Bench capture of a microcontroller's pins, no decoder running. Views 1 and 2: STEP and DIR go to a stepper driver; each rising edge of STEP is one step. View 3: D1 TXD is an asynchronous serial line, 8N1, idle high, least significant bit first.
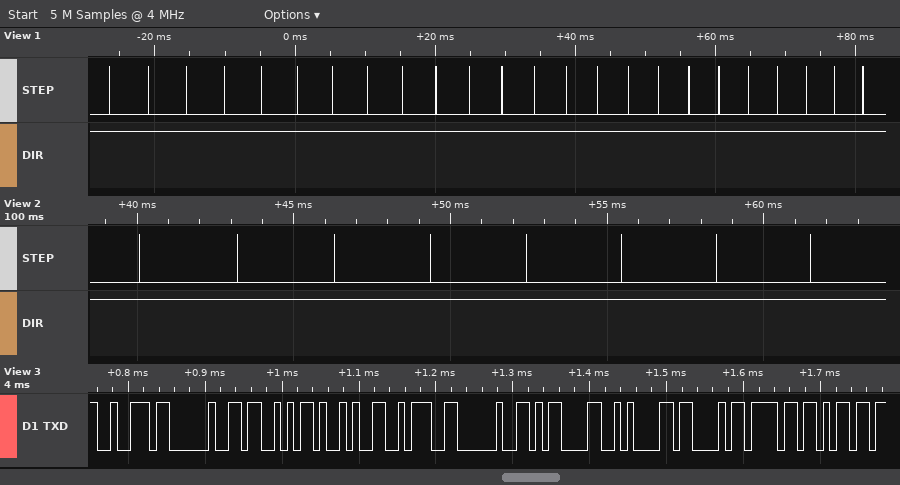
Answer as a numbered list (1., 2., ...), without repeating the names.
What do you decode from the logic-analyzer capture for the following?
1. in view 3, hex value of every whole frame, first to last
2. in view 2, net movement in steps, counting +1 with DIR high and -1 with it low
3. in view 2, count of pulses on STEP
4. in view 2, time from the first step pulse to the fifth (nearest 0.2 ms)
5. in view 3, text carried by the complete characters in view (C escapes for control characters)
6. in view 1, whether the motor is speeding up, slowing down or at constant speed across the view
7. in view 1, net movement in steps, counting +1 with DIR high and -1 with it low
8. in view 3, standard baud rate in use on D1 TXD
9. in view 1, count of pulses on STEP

1. 0x72 0x20 0x53 0x29 0x3A 0x20 0x0D 0x0A 0x43 0x6F 0x6D
2. +8
3. 8
4. 12.4 ms
5. "r S): \r\nCom"
6. speeding up
7. +24
8. 115200 baud
9. 24
